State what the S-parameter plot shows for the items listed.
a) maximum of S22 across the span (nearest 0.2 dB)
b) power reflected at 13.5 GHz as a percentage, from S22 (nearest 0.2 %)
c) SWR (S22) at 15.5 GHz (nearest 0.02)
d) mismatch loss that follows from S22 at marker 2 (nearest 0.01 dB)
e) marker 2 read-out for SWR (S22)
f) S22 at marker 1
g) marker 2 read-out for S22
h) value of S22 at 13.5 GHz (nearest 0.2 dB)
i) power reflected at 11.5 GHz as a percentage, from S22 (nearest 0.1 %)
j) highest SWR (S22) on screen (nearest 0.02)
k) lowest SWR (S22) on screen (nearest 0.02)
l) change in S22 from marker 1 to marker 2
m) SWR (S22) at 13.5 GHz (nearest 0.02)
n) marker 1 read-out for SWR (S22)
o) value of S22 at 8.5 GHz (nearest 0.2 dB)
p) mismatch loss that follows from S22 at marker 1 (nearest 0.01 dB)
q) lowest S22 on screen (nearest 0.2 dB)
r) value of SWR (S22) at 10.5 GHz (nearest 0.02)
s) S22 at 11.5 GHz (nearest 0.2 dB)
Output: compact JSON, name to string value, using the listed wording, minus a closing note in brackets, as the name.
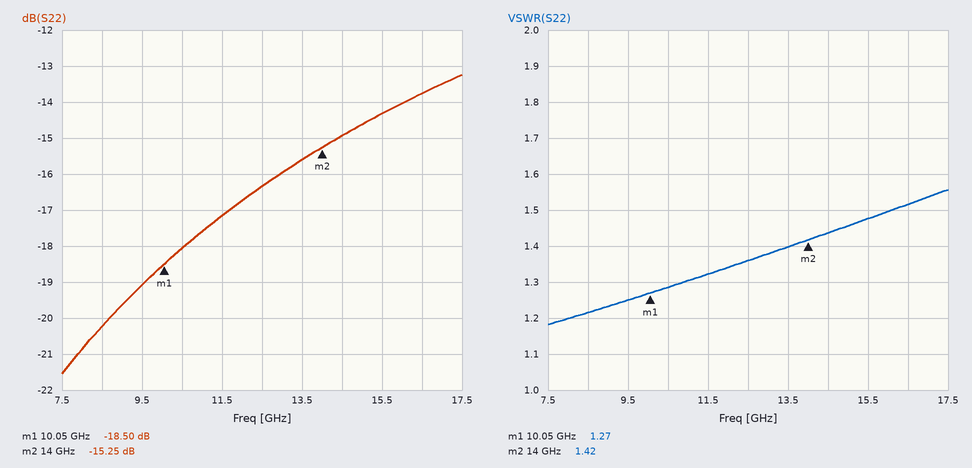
{"maximum of S22 across the span": "-13.2 dB", "power reflected at 13.5 GHz as a percentage, from S22": "2.8 %", "SWR (S22) at 15.5 GHz": "1.48", "mismatch loss that follows from S22 at marker 2": "0.13 dB", "marker 2 read-out for SWR": "1.42", "S22 at marker 1": "-18.50 dB", "marker 2 read-out for S22": "-15.25 dB", "value of S22 at 13.5 GHz": "-15.6 dB", "power reflected at 11.5 GHz as a percentage, from S22": "1.9 %", "highest SWR (S22) on screen": "1.56", "lowest SWR (S22) on screen": "1.18", "change in S22 from marker 1 to marker 2": "3.25 dB", "SWR (S22) at 13.5 GHz": "1.40", "marker 1 read-out for SWR": "1.27", "value of S22 at 8.5 GHz": "-20.2 dB", "mismatch loss that follows from S22 at marker 1": "0.06 dB", "lowest S22 on screen": "-21.6 dB", "value of SWR (S22) at 10.5 GHz": "1.28", "S22 at 11.5 GHz": "-17.2 dB"}
